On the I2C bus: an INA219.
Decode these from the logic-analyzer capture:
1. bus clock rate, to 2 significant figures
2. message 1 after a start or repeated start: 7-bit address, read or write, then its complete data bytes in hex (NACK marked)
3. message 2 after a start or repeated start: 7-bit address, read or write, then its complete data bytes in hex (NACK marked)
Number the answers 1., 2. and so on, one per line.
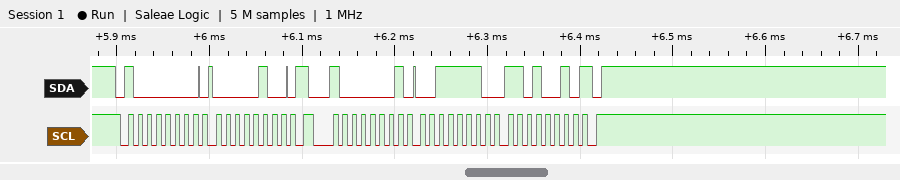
1. 100 kHz
2. 0x40 write: 04
3. 0x40 read: 3E D2 NACK
